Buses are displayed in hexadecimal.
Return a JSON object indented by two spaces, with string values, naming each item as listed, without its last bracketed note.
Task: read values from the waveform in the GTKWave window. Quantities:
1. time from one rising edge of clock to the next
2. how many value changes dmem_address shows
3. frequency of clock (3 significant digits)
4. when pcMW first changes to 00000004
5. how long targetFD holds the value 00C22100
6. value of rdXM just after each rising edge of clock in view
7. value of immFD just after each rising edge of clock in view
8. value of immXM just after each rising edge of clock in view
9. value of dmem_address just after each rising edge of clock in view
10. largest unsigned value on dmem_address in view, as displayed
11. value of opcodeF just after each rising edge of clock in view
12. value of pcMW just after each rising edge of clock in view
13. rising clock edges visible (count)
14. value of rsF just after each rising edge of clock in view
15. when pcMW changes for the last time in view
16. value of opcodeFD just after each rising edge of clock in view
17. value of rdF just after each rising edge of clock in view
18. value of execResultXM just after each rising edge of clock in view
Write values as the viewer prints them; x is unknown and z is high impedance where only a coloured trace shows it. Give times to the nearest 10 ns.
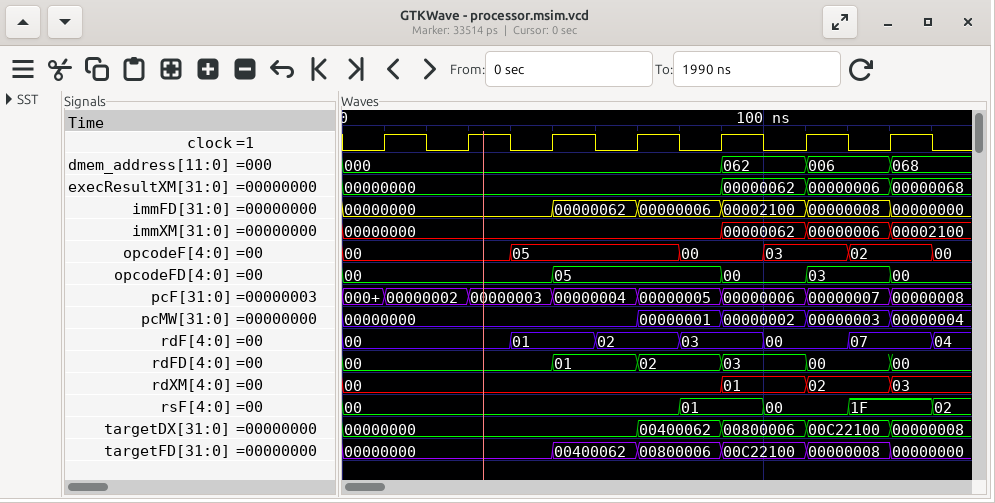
{
  "time from one rising edge of clock to the next": "20 ns",
  "how many value changes dmem_address shows": "3",
  "frequency of clock": "50.0 MHz",
  "when pcMW first changes to 00000004": "130 ns",
  "how long targetFD holds the value 00C22100": "20 ns",
  "value of rdXM just after each rising edge of clock in view": "00, 00, 00, 00, 01, 02, 03",
  "value of immFD just after each rising edge of clock in view": "00000000, 00000000, 00000062, 00000006, 00002100, 00000008, 00000000",
  "value of immXM just after each rising edge of clock in view": "00000000, 00000000, 00000000, 00000000, 00000062, 00000006, 00002100",
  "value of dmem_address just after each rising edge of clock in view": "000, 000, 000, 000, 062, 006, 068",
  "largest unsigned value on dmem_address in view, as displayed": "068",
  "value of opcodeF just after each rising edge of clock in view": "00, 00, 05, 05, 00, 03, 02",
  "value of pcMW just after each rising edge of clock in view": "00000000, 00000000, 00000000, 00000001, 00000002, 00000003, 00000004",
  "rising clock edges visible": "7",
  "value of rsF just after each rising edge of clock in view": "00, 00, 00, 00, 01, 00, 1F",
  "when pcMW changes for the last time in view": "130 ns",
  "value of opcodeFD just after each rising edge of clock in view": "00, 00, 05, 05, 00, 03, 00",
  "value of rdF just after each rising edge of clock in view": "00, 00, 01, 02, 03, 00, 07",
  "value of execResultXM just after each rising edge of clock in view": "00000000, 00000000, 00000000, 00000000, 00000062, 00000006, 00000068"
}
